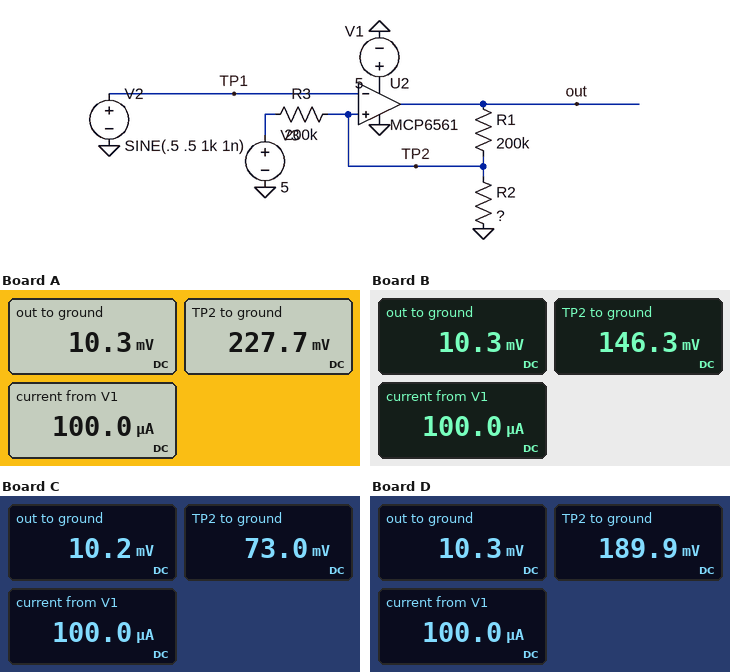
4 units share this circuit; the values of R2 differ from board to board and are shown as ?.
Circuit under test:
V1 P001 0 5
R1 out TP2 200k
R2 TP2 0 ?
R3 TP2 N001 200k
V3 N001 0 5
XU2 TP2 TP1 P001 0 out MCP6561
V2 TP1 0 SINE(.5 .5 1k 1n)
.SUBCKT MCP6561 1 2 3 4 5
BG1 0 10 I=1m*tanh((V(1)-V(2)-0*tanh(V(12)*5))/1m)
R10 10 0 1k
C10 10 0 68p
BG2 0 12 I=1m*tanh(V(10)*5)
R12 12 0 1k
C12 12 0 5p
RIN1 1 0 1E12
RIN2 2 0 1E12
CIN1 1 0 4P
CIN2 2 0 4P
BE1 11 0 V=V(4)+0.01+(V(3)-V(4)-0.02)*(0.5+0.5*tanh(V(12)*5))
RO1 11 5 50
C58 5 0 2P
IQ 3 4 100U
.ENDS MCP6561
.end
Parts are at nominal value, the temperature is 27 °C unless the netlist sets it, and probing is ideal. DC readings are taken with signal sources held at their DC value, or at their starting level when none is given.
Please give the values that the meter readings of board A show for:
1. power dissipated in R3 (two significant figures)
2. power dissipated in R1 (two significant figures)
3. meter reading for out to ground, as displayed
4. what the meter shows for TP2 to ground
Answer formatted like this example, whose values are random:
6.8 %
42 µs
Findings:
110 µW
240 nW
10.3 mV
227.7 mV
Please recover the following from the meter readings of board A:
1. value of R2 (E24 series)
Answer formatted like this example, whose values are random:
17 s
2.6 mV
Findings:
10 kΩ
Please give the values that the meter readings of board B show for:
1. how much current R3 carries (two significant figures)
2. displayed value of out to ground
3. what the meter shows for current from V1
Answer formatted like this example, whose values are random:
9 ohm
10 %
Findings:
24 µA
10.3 mV
100.0 µA
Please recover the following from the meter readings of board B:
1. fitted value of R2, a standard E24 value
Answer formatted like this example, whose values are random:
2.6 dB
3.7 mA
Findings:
6.2 kΩ
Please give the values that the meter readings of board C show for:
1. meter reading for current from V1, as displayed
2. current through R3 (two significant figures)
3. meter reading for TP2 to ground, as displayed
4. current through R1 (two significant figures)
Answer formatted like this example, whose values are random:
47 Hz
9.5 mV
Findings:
100.0 µA
25 µA
73.0 mV
310 nA
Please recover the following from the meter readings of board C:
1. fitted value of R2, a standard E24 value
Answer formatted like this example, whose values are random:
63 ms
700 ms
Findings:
3 kΩ
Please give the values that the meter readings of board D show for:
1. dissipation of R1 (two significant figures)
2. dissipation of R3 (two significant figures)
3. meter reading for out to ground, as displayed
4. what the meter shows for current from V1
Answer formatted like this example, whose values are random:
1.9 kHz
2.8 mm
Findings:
160 nW
120 µW
10.3 mV
100.0 µA
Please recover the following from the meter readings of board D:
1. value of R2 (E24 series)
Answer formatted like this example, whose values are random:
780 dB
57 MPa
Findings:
8.2 kΩ
